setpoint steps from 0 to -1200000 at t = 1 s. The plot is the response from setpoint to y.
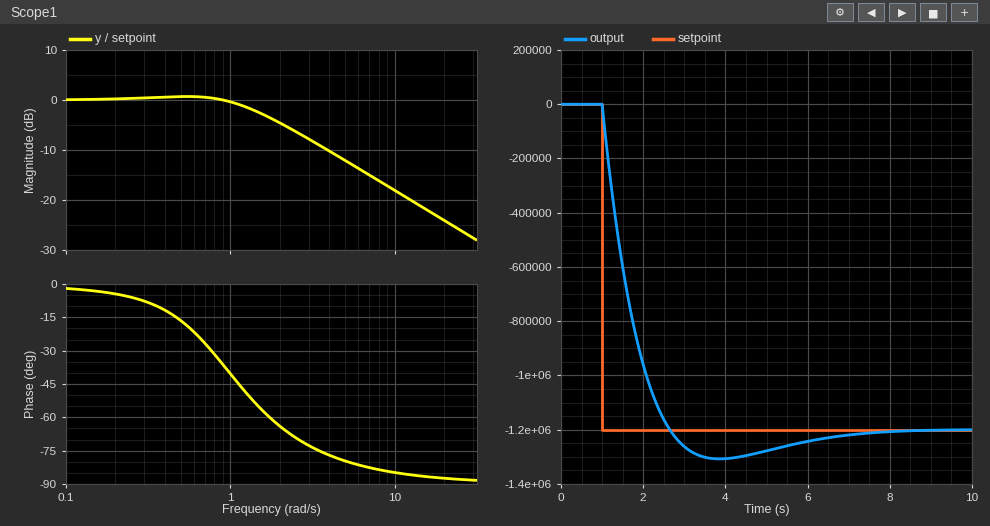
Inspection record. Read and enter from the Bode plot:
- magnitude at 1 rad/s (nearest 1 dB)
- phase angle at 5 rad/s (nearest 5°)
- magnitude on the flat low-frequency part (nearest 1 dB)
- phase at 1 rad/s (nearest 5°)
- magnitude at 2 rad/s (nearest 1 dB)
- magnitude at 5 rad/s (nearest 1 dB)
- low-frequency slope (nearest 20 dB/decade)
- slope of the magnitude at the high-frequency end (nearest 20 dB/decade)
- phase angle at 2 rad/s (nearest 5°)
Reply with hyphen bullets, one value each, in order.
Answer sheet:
- 0 dB
- -80°
- 0 dB
- -40°
- -5 dB
- -12 dB
- 0 dB/decade
- -20 dB/decade
- -65°
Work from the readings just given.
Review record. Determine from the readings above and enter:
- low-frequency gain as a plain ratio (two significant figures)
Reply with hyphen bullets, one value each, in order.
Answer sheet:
- 1.0
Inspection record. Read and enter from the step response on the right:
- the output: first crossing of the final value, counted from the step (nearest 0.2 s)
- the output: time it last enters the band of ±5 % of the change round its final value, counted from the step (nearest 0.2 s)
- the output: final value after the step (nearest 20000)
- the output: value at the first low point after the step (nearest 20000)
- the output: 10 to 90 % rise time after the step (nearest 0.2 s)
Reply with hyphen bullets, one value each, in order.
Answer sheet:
- 1.6 s
- 4.4 s
- -1200000
- -1300000
- 1.2 s
